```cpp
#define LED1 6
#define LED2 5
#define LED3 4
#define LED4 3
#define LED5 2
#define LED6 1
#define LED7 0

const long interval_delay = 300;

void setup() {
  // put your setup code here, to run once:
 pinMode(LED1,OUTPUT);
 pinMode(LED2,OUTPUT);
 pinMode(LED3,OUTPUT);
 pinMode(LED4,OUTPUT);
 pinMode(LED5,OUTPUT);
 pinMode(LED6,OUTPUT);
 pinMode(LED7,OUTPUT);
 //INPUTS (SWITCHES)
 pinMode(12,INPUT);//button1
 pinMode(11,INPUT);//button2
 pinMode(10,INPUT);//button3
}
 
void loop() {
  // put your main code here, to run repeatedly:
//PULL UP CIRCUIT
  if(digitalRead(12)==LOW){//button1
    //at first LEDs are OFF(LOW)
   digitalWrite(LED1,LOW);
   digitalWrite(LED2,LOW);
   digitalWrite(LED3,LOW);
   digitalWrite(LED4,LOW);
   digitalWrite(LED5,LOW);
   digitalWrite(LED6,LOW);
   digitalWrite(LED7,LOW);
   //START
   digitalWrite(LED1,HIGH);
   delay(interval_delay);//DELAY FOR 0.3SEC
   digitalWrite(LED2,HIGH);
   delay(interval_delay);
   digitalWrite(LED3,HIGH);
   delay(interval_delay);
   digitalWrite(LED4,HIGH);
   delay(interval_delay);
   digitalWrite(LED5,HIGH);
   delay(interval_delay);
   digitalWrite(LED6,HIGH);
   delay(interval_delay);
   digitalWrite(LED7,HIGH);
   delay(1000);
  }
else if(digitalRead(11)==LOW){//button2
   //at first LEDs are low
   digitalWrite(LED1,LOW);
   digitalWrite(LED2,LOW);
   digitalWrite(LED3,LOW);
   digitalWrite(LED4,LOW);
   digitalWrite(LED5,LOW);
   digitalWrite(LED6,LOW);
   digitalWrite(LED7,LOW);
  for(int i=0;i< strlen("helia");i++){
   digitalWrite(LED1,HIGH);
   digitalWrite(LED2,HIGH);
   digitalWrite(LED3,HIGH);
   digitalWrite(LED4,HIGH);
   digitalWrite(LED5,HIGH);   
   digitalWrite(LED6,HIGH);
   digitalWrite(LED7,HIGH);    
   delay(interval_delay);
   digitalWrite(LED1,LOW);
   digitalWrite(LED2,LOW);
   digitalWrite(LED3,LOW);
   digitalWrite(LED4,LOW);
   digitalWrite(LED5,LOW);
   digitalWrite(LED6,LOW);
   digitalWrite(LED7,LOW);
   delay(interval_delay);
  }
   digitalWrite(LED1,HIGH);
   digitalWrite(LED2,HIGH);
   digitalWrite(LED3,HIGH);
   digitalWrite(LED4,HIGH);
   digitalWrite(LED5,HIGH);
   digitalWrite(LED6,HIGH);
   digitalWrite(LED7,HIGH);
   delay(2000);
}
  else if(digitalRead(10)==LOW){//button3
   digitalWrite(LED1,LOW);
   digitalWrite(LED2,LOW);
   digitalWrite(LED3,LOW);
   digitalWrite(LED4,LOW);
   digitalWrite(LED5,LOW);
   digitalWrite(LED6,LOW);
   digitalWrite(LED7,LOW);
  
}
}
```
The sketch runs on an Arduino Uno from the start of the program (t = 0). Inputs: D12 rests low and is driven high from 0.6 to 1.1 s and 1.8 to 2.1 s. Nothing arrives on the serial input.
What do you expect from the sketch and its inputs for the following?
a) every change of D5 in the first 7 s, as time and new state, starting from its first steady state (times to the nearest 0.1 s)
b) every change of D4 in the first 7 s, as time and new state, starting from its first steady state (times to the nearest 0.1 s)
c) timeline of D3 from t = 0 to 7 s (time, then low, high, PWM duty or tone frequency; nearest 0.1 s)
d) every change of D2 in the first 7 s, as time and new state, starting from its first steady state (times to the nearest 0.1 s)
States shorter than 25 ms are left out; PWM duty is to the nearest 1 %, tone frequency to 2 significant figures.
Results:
0 s low; 0.3 s high; 2.8 s low; 3.1 s high; 5.6 s low; 5.9 s high
0 s low; 0.6 s high; 2.8 s low; 3.4 s high; 5.6 s low; 6.2 s high
0 s low; 0.9 s high; 2.8 s low; 3.7 s high; 5.6 s low; 6.5 s high
0 s low; 1.2 s high; 2.8 s low; 4 s high; 5.6 s low; 6.8 s high
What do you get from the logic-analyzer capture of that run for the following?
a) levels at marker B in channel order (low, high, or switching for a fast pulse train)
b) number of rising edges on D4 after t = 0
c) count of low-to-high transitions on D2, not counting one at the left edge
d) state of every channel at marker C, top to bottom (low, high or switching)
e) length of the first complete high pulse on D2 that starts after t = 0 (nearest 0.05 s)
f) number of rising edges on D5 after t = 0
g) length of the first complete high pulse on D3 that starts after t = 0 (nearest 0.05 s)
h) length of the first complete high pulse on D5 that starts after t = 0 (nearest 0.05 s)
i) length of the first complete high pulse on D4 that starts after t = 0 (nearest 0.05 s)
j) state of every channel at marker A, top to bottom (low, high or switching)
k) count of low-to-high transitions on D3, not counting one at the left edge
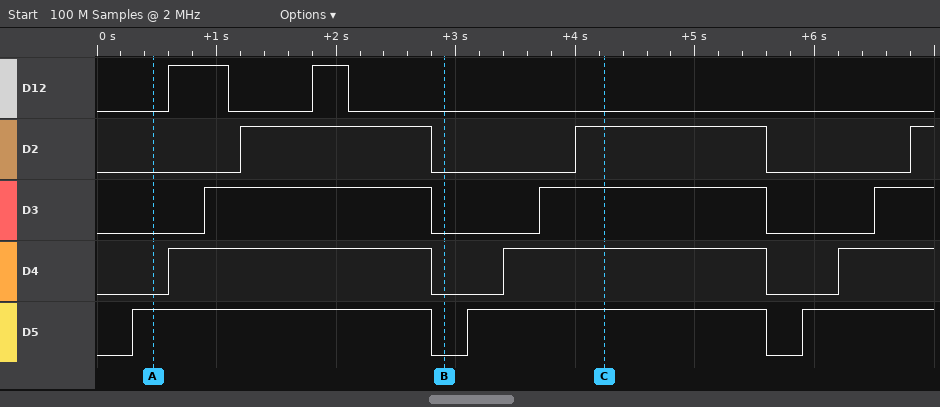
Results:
D12 low, D2 low, D3 low, D4 low, D5 low
3
3
D12 low, D2 high, D3 high, D4 high, D5 high
1.60 s
3
1.90 s
2.50 s
2.20 s
D12 low, D2 low, D3 low, D4 low, D5 high
3
